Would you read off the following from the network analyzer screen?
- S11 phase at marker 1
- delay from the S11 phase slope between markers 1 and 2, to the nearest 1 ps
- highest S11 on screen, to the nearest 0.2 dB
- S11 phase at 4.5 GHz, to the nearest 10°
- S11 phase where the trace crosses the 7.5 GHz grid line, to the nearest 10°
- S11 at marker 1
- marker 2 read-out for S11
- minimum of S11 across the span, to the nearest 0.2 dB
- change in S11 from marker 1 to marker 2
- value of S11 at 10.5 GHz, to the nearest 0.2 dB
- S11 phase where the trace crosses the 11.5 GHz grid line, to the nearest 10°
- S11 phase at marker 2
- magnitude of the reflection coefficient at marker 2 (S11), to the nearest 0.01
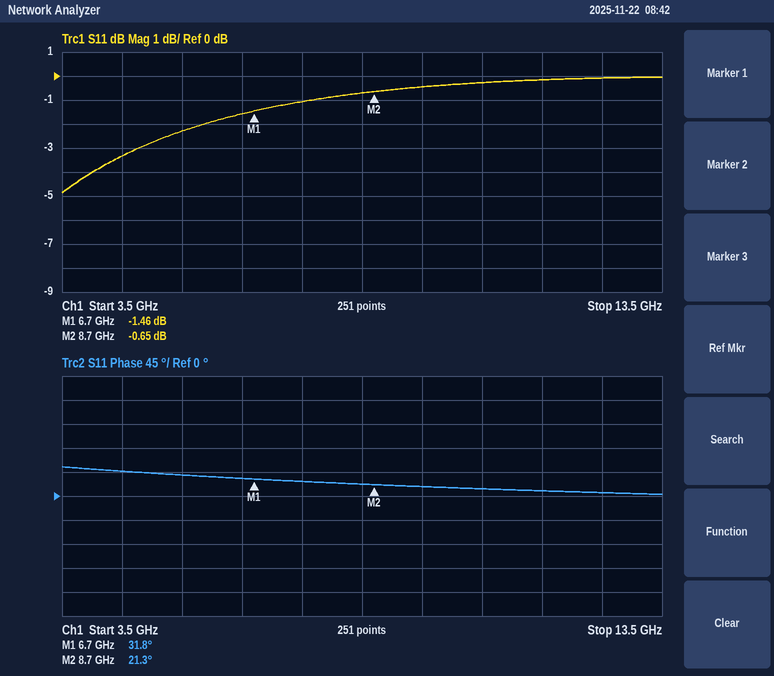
31.8°
15 ps
0.0 dB
50°
30°
-1.46 dB
-0.65 dB
-4.8 dB
0.81 dB
-0.2 dB
10°
21.3°
0.93
